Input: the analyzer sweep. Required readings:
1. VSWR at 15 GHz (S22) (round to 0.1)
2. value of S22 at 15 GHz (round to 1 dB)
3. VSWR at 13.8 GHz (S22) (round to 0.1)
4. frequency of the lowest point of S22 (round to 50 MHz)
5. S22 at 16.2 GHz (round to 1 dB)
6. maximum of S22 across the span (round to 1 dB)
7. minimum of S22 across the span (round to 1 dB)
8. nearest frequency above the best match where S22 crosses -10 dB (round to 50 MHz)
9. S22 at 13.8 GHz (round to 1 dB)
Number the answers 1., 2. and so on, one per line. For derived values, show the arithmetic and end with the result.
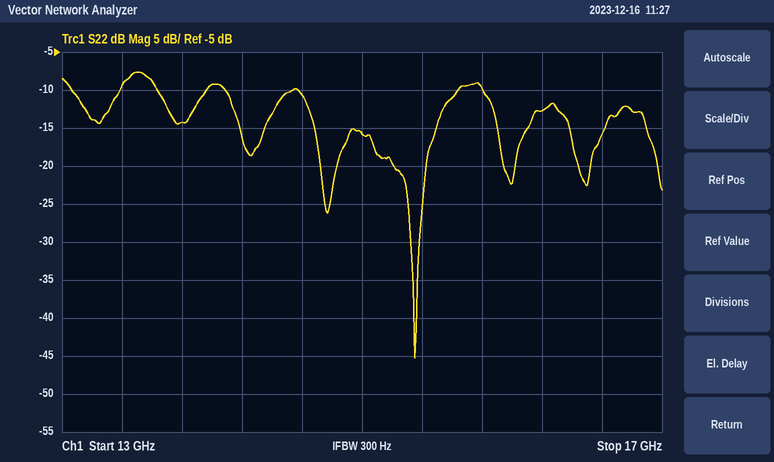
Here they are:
1. |Γ| = 10^(-16/20) = 0.1585; VSWR = (1 + 0.1585)/(1 − 0.1585) ≈ 1.4
2. -16 dB
3. |Γ| = 10^(-14/20) = 0.1995; VSWR = (1 + 0.1995)/(1 − 0.1995) ≈ 1.5
4. 15.35 GHz
5. -13 dB
6. -8 dB
7. -45 dB
8. 15.65 GHz
9. -14 dB
